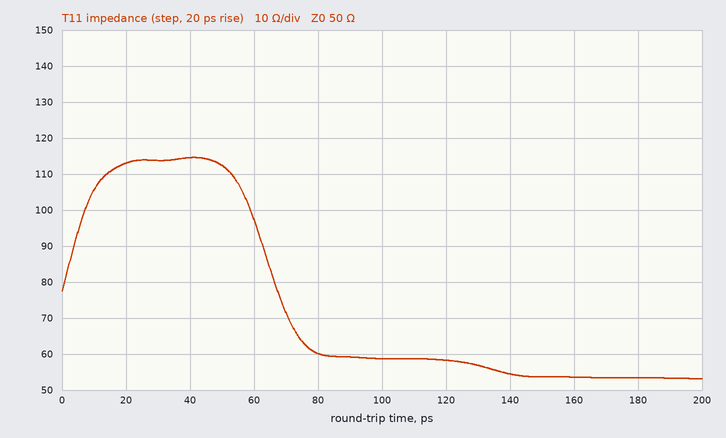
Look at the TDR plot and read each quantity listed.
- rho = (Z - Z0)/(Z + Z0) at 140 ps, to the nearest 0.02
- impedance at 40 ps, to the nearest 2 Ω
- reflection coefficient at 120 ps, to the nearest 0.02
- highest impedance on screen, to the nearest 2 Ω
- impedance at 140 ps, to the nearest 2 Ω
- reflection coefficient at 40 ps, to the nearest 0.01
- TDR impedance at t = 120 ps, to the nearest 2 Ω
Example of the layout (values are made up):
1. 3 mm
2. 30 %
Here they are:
1. +0.04
2. 114 Ω
3. +0.08
4. 114 Ω
5. 54 Ω
6. +0.39
7. 58 Ω
